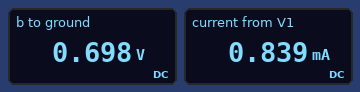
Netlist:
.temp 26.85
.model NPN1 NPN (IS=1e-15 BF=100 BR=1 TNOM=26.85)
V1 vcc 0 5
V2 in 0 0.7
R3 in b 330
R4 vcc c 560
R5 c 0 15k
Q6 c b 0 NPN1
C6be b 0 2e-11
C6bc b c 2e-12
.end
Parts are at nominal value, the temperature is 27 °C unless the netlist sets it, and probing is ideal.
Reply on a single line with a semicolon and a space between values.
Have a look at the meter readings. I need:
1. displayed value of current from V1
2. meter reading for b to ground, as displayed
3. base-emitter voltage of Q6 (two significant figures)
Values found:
0.839 mA; 0.698 V; 700 mV
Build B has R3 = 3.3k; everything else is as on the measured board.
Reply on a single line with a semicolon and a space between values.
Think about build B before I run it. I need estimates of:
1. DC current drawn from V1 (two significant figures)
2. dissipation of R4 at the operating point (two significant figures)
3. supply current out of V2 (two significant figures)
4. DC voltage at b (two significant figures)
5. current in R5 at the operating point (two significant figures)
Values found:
670 µA; 250 µW; 3.6 µA; 690 mV; 310 µA
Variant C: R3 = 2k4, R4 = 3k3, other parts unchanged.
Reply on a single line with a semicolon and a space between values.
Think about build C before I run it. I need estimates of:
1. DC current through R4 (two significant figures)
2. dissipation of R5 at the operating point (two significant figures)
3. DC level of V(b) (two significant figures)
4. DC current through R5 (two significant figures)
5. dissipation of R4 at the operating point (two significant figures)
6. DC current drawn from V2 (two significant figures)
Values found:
600 µA; 610 µW; 690 mV; 200 µA; 1.2 mW; 4.0 µA
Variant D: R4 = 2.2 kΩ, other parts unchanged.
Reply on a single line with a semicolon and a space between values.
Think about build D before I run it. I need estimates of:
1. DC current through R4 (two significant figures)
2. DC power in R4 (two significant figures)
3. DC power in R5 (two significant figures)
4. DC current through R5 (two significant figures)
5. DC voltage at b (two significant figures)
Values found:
760 µA; 1.3 mW; 740 µW; 220 µA; 700 mV
